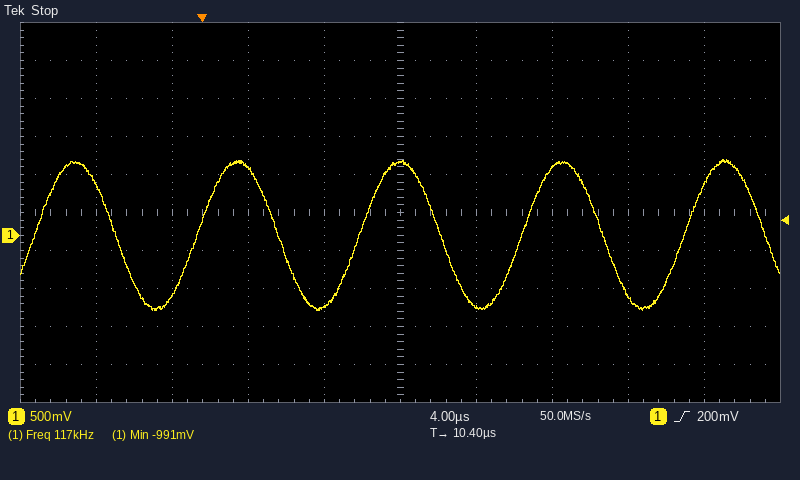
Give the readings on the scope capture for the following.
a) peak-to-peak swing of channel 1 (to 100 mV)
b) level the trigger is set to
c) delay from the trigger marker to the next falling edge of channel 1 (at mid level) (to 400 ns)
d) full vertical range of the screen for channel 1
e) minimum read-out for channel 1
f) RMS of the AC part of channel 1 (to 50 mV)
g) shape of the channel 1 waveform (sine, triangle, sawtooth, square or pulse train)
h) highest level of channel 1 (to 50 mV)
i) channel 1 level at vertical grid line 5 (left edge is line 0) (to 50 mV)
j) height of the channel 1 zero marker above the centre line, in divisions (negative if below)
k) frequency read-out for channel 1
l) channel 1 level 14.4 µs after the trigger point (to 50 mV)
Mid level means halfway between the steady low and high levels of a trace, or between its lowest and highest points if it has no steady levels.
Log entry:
2.00 V
200 mV
4.0 µs
5 V
-991 mV
700 mV
sine
1.00 V
950 mV
-0.6 div
117 kHz
-950 mV
